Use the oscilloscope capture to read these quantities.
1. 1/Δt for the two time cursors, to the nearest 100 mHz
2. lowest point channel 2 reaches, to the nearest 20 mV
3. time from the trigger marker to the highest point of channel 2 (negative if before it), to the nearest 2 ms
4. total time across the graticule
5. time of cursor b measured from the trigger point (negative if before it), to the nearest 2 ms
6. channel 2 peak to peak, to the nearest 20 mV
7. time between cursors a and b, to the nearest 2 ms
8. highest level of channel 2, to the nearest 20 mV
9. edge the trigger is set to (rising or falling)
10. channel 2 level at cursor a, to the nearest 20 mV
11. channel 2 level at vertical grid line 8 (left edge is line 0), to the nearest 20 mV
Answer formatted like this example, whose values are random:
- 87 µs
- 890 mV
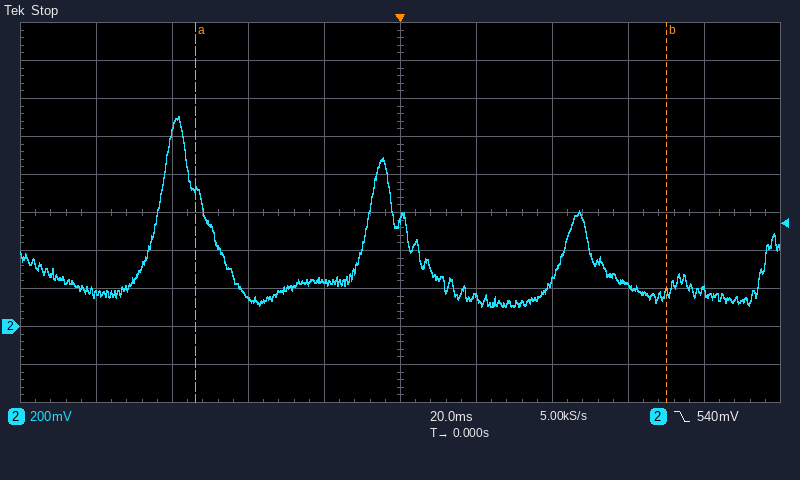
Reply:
- 8.1 Hz
- 100 mV
- -58 ms
- 200 ms
- +70 ms
- 1.00 V
- 124 ms
- 1.10 V
- falling
- 720 mV
- 220 mV
